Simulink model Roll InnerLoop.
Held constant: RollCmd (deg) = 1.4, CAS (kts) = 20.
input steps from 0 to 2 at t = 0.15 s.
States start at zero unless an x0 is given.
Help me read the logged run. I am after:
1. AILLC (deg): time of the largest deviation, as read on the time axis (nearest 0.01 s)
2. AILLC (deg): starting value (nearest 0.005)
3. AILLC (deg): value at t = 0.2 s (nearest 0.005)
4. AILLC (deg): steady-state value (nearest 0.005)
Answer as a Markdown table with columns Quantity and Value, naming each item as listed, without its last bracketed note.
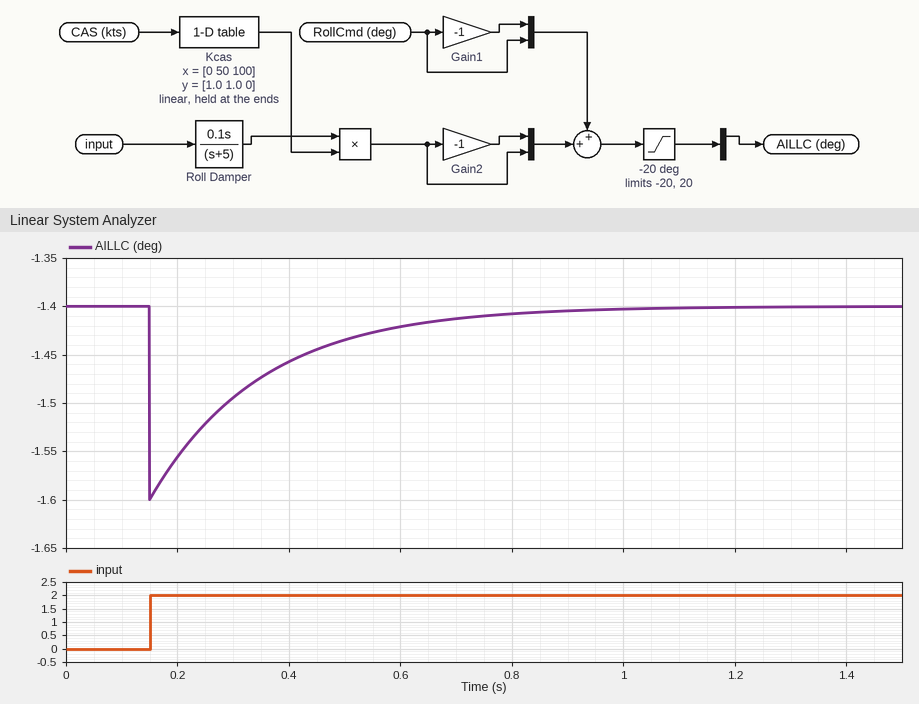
| Quantity | Value |
|---|---|
| AILLC (deg): time of the largest deviation, as read on the time axis | 0.15 s |
| AILLC (deg): starting value | -1.400 |
| AILLC (deg): value at t = 0.2 s | -1.555 |
| AILLC (deg): steady-state value | -1.400 |
